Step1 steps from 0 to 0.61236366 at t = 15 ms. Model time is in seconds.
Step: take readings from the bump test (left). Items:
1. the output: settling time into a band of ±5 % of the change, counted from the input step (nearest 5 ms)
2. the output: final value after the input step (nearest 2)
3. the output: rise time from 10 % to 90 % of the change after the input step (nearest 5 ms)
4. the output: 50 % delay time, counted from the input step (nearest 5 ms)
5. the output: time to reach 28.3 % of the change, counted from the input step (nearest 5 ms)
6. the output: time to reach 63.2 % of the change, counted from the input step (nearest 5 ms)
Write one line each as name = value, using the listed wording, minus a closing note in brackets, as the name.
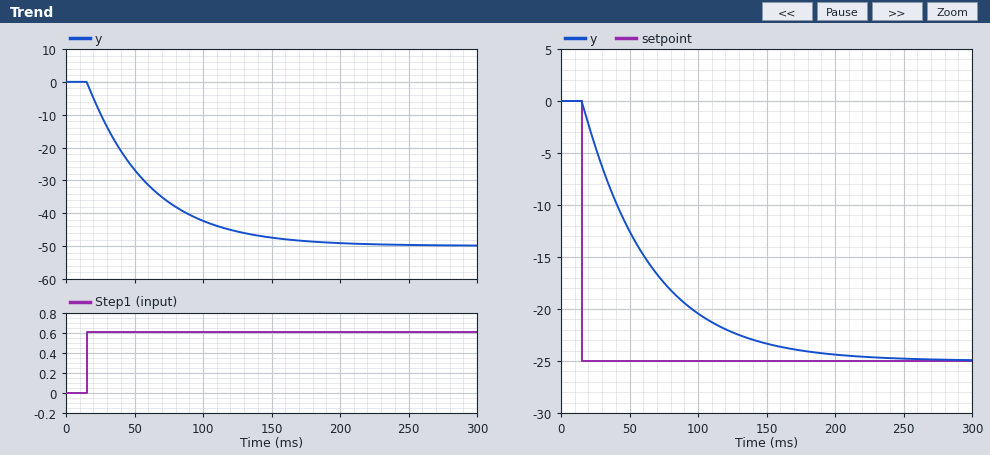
the output: settling time into a band of ±5 % of the change, counted from the input step = 135 ms
the output: final value after the input step = -50
the output: rise time from 10 % to 90 % of the change after the input step = 100 ms
the output: 50 % delay time, counted from the input step = 30 ms
the output: time to reach 28.3 % of the change, counted from the input step = 15 ms
the output: time to reach 63.2 % of the change, counted from the input step = 45 ms
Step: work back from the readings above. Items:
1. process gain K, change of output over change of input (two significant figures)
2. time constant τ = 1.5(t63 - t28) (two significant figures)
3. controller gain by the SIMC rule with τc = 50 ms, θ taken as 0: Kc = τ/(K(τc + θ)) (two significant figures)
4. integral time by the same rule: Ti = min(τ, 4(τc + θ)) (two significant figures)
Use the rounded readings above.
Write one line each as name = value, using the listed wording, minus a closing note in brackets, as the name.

process gain K, change of output over change of input = -82
time constant τ = 1.5(t63 - t28) = 45 ms
controller gain by the SIMC rule with τc = 50 ms, θ taken as 0: Kc = τ/(K(τc + θ)) = -0.011
integral time by the same rule: Ti = min(τ, 4(τc + θ)) = 45 ms
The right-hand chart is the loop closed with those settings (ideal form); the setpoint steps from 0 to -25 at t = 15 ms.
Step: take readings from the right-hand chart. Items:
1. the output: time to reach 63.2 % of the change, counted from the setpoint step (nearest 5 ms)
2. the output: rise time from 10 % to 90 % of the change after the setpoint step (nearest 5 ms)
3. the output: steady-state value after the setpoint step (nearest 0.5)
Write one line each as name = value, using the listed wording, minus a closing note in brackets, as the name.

the output: time to reach 63.2 % of the change, counted from the setpoint step = 50 ms
the output: rise time from 10 % to 90 % of the change after the setpoint step = 110 ms
the output: steady-state value after the setpoint step = -25.0
